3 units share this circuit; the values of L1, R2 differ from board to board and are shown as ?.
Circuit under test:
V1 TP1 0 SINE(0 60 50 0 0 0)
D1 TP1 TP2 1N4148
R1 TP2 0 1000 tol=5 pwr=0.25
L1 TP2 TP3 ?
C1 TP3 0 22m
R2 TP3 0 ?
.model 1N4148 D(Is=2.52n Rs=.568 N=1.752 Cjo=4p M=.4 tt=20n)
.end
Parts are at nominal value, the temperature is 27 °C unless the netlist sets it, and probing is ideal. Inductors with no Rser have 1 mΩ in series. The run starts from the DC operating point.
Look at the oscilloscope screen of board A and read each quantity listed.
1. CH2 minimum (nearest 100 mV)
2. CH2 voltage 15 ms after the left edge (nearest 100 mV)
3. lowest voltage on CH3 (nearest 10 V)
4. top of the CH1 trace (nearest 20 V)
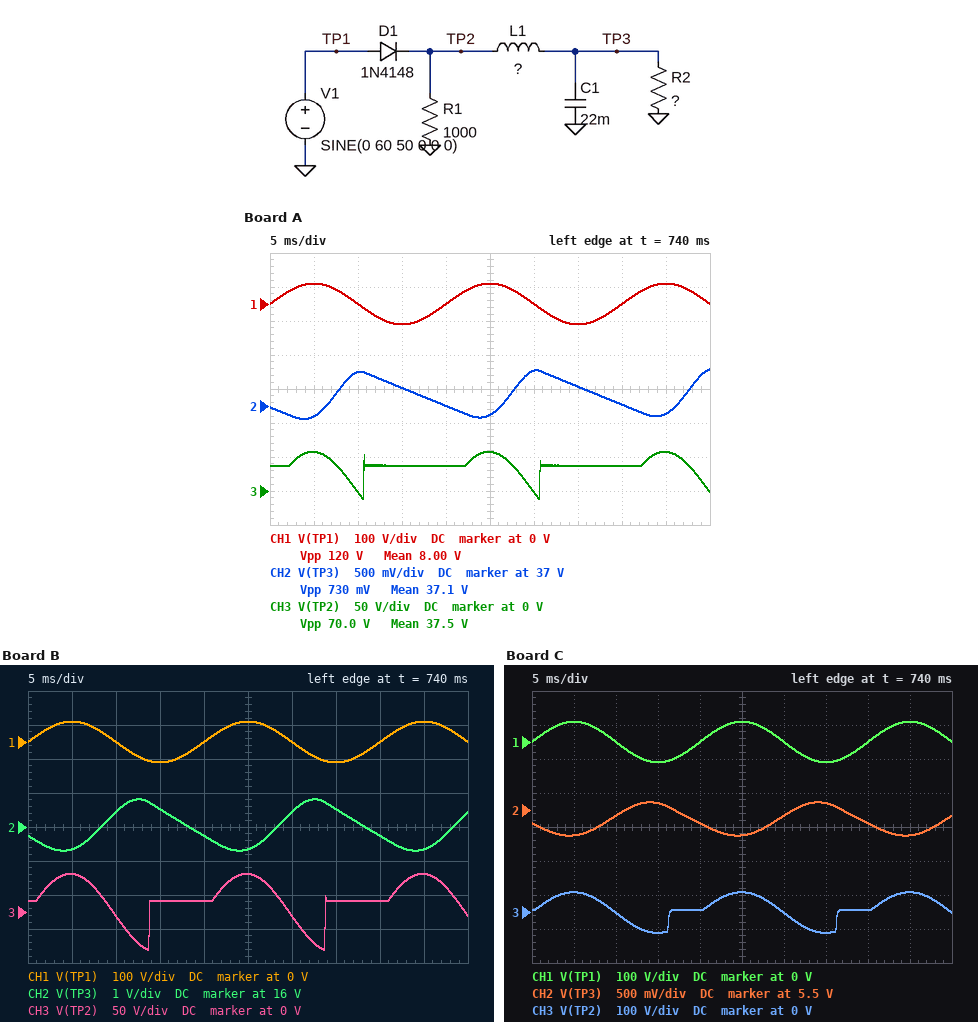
36.8 V
37.3 V
-10 V
60 V
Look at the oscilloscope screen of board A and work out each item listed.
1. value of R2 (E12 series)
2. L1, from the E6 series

33 Ω
15 mH
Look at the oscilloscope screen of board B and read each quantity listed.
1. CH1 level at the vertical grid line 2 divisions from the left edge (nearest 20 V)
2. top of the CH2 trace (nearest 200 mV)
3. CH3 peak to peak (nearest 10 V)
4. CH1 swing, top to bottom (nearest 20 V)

0 V
16.8 V
110 V
120 V
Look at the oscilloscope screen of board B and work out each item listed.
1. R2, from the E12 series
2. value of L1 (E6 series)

4.7 Ω
22 mH
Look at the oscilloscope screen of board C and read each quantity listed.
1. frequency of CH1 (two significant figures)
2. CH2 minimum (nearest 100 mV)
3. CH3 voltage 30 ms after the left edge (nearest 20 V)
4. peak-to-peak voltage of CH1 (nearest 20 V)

50 Hz
5.1 V
0 V
120 V
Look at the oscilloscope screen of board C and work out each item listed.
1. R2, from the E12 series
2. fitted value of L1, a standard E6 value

3.9 Ω
100 mH
